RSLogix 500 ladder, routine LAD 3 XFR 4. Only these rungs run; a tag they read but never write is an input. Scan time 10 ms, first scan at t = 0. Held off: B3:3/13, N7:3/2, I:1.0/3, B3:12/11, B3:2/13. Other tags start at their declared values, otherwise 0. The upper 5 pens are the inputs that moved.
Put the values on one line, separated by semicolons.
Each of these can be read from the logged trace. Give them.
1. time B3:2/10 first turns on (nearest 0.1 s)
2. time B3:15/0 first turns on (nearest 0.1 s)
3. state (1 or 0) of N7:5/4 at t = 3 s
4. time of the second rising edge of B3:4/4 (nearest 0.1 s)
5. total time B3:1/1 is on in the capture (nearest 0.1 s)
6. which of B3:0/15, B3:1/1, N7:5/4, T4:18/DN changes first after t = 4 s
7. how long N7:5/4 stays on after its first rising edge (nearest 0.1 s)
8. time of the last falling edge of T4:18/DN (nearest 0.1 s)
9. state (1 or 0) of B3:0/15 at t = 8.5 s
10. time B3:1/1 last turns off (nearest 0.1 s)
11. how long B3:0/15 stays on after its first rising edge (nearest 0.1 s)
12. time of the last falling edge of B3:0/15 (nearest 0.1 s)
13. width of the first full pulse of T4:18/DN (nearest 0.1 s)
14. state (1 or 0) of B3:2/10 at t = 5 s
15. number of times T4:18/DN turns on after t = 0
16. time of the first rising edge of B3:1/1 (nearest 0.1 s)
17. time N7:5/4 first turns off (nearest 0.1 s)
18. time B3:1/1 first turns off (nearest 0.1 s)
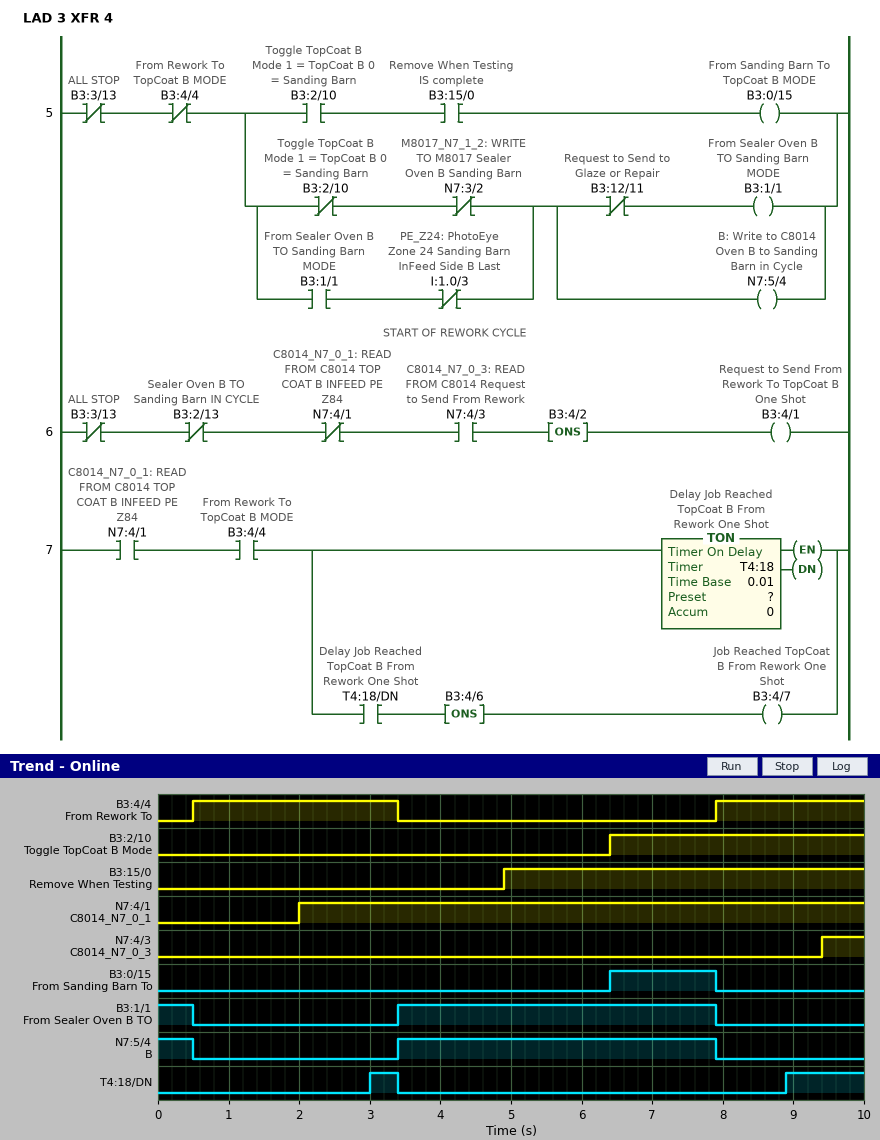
6.4 s; 4.9 s; 0; 7.9 s; 5.0 s; B3:0/15; 4.5 s; 3.4 s; 0; 7.9 s; 1.5 s; 7.9 s; 0.4 s; 0; 2; 3.4 s; 0.5 s; 0.5 s
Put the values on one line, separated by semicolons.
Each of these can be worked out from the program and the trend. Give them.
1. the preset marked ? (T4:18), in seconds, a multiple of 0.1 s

1.0 s
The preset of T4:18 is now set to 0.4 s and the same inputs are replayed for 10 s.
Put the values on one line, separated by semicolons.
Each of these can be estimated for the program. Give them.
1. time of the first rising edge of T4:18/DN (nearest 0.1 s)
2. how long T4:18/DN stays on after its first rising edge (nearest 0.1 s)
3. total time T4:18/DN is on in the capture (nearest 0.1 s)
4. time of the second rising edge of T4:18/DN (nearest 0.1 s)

2.4 s; 1.0 s; 2.7 s; 8.3 s
